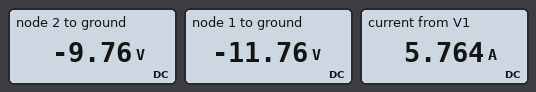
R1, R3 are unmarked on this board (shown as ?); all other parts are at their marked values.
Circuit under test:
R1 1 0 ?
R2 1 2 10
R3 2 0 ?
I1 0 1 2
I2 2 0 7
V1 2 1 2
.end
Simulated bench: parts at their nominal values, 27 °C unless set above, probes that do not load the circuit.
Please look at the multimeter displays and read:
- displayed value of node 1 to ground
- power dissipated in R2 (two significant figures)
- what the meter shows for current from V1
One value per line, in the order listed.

-11.76 V
400 mW
5.764 A
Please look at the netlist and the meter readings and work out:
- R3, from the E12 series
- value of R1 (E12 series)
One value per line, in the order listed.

6.8 Ω
3.3 Ω
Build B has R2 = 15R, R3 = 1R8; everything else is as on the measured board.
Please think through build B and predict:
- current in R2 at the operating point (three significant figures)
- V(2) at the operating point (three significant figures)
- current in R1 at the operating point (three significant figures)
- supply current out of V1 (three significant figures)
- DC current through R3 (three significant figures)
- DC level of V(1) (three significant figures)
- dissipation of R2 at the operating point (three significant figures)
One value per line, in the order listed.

133 mA
-5.12 V
2.16 A
4.29 A
2.84 A
-7.12 V
267 mW
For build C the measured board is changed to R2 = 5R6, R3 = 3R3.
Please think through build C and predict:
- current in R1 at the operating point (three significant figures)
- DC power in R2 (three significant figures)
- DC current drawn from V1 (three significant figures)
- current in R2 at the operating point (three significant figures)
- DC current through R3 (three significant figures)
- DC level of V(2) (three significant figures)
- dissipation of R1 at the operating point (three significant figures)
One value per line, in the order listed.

2.80 A
714 mW
5.16 A
357 mA
2.20 A
-7.25 V
25.9 W
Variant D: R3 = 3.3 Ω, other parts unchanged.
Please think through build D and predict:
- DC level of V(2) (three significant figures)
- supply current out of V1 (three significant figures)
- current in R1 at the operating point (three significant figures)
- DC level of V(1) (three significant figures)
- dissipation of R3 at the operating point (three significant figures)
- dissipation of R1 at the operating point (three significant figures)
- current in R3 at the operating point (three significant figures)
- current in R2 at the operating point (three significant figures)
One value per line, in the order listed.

-7.25 V
5.00 A
2.80 A
-9.25 V
15.9 W
25.9 W
2.20 A
200 mA
